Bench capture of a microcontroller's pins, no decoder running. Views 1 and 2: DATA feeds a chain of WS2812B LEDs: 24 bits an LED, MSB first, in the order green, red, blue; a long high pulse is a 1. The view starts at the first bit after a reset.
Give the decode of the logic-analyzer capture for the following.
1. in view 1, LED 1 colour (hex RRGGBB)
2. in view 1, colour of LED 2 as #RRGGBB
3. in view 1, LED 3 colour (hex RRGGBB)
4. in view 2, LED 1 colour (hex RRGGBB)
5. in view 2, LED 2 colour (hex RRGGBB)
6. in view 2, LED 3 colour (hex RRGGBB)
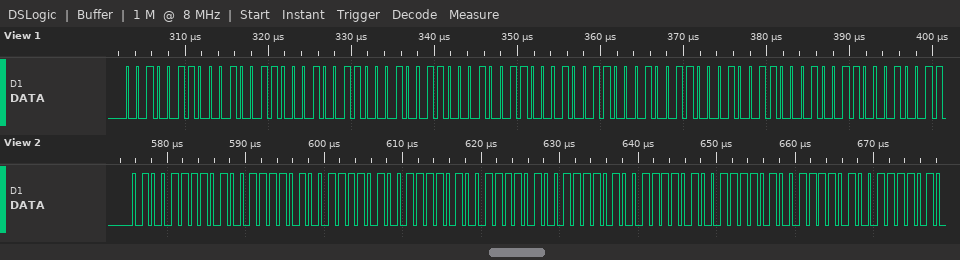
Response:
#262626
#262626
#262626
#4F4F4F
#4F4F4F
#4F4F4F
